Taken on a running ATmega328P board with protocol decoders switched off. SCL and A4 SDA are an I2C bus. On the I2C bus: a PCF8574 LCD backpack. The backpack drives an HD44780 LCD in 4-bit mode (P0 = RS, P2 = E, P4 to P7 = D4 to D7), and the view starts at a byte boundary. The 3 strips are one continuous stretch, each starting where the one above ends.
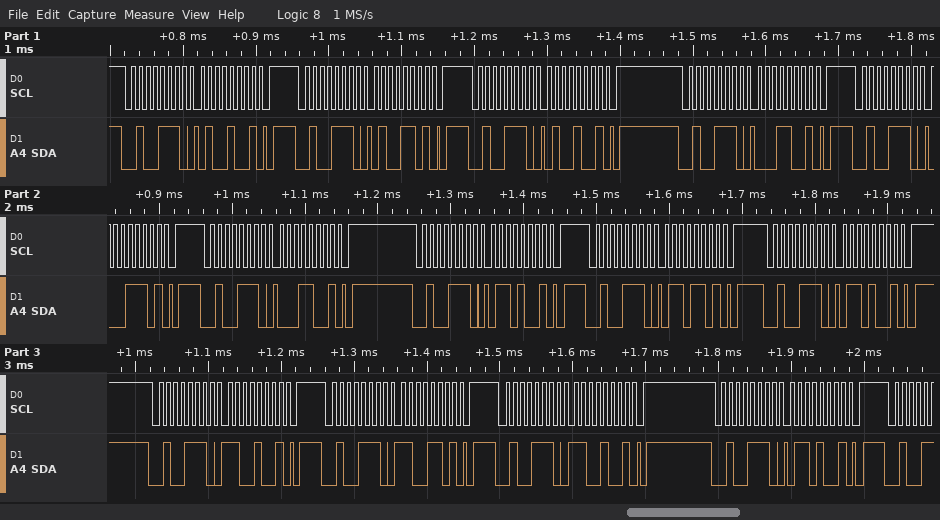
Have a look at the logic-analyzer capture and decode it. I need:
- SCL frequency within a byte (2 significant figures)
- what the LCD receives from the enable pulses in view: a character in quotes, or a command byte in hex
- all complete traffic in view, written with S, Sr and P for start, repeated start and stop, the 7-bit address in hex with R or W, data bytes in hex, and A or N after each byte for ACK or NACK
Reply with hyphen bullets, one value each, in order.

- 100 kHz
- 'A' 'l'
- S 27W A 49 A P S 27W A 4D A P S 27W A 49 A P S 27W A 19 A P S 27W A 1D A P S 27W A 19 A P S 27W A 69 A P S 27W A 6D A P S 27W A 69 A P S 27W A C9 A P S 27W A CD A P S 27W A C9 A P S 27W A 69 A P
